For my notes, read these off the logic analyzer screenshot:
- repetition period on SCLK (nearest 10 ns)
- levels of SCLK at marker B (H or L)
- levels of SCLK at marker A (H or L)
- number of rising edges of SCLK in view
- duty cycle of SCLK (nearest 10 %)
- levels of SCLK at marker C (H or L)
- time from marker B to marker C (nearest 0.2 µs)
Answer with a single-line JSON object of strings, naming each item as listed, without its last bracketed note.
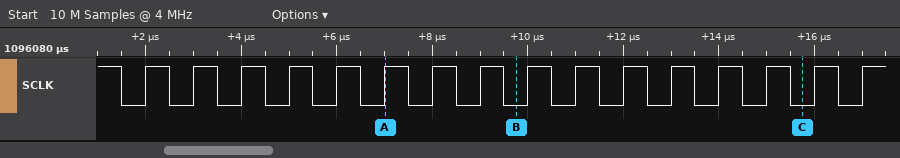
{"repetition period on SCLK": "1000 ns", "levels of SCLK at marker B": "SCLK=L", "levels of SCLK at marker A": "SCLK=H", "number of rising edges of SCLK in view": "16", "duty cycle of SCLK": "50 %", "levels of SCLK at marker C": "SCLK=L", "time from marker B to marker C": "6 µs"}
